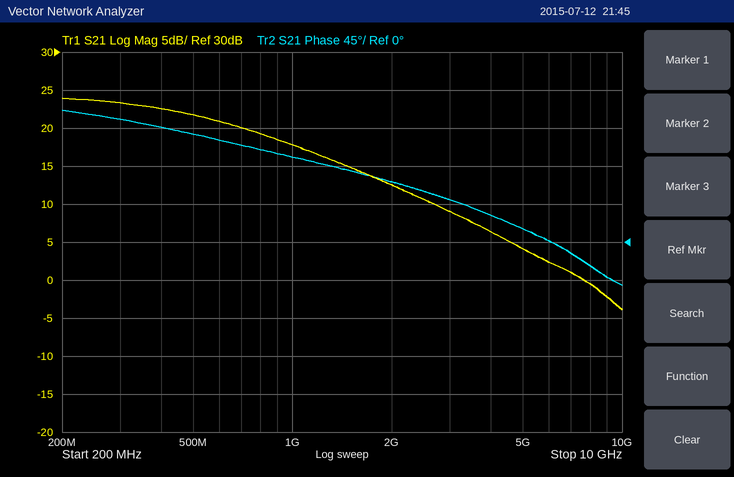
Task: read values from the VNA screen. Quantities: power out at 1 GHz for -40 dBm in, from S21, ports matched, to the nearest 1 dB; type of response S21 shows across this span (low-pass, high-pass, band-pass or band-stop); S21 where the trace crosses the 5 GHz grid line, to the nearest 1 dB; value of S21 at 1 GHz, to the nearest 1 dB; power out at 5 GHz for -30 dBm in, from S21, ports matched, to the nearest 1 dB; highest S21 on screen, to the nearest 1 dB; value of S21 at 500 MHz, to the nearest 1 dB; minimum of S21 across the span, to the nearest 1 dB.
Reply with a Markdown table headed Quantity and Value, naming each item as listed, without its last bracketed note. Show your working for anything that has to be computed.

| Quantity | Value |
|---|---|
| power out at 1 GHz for -40 dBm in, from S21, ports matched, to the nearest 1 dB | -40 dBm + (18 dB) = -22 dBm |
| type of response S21 shows across this span | low-pass |
| S21 where the trace crosses the 5 GHz grid line, to the nearest 1 dB | 4 dB |
| value of S21 at 1 GHz, to the nearest 1 dB | 18 dB |
| power out at 5 GHz for -30 dBm in, from S21, ports matched, to the nearest 1 dB | -30 dBm + (4 dB) = -26 dBm |
| highest S21 on screen, to the nearest 1 dB | 24 dB |
| value of S21 at 500 MHz, to the nearest 1 dB | 22 dB |
| minimum of S21 across the span, to the nearest 1 dB | -4 dB |
